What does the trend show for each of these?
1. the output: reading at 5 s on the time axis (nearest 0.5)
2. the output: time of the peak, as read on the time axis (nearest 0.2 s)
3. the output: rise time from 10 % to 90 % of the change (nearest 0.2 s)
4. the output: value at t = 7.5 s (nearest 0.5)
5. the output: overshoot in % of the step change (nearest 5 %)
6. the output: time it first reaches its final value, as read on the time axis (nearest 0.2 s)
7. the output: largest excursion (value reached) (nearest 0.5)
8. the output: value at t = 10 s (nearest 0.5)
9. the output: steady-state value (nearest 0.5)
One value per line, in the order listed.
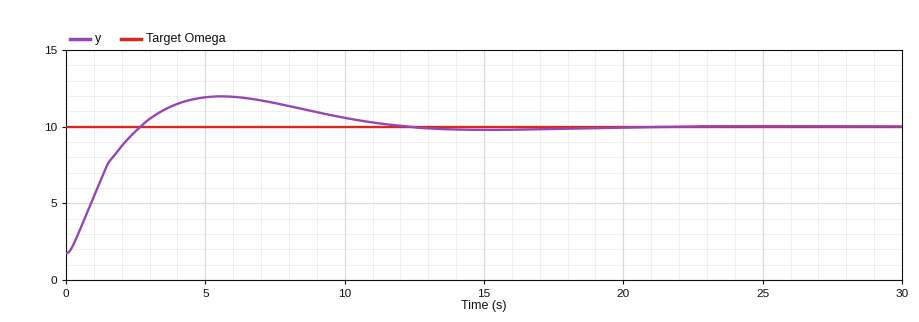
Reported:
12.0
5.6 s
1.8 s
11.5
25 %
2.6 s
12.0
10.5
10.0
